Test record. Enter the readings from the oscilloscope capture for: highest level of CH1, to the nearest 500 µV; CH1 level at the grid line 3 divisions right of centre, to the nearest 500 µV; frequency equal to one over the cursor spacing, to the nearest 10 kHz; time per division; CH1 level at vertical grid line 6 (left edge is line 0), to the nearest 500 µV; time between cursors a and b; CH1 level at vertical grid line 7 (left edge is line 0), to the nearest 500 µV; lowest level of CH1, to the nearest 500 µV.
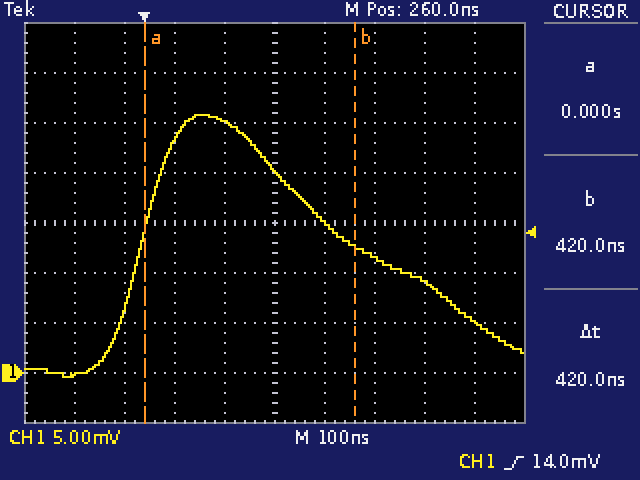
26.0 mV
9.0 mV
2.38 MHz
100 ns
15.0 mV
420 ns
11.5 mV
-500 µV
